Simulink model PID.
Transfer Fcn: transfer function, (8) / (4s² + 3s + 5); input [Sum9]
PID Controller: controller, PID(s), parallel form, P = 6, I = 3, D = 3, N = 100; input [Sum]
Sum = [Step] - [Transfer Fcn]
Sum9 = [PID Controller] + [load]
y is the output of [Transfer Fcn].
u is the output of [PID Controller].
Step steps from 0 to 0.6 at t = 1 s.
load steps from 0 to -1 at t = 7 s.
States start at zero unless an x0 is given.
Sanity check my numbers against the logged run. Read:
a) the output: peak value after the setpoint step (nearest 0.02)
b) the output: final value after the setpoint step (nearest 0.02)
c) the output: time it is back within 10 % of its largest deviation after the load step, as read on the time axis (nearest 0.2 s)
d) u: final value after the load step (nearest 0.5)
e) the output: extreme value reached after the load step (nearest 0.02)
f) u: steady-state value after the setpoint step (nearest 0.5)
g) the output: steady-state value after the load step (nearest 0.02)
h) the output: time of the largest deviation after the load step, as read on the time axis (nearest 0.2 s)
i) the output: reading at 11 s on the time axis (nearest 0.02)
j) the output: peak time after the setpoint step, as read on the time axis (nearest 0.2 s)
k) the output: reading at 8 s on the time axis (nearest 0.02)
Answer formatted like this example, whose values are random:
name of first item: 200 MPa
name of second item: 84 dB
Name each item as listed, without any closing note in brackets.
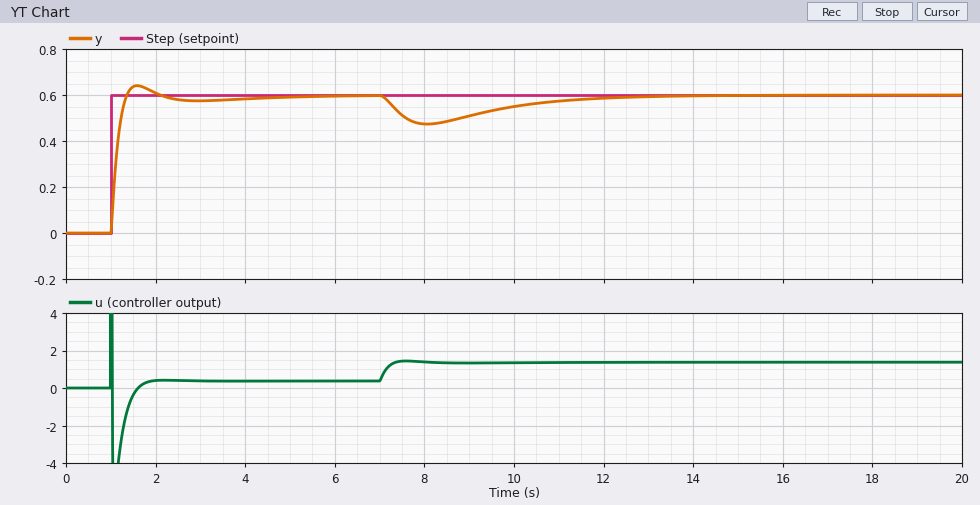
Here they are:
the output: peak value after the setpoint step: 0.64
the output: final value after the setpoint step: 0.60
the output: time it is back within 10 % of its largest deviation after the load step, as read on the time axis: 12.2 s
u: final value after the load step: 1.5
the output: extreme value reached after the load step: 0.48
u: steady-state value after the setpoint step: 0.5
the output: steady-state value after the load step: 0.60
the output: time of the largest deviation after the load step, as read on the time axis: 8.0 s
the output: reading at 11 s on the time axis: 0.58
the output: peak time after the setpoint step, as read on the time axis: 1.6 s
the output: reading at 8 s on the time axis: 0.48
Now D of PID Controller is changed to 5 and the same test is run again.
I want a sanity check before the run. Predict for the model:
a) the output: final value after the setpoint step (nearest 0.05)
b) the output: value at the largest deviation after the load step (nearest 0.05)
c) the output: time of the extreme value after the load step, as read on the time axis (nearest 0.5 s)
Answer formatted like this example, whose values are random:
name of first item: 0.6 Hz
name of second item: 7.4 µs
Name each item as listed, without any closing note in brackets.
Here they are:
the output: final value after the setpoint step: 0.60
the output: value at the largest deviation after the load step: 0.50
the output: time of the extreme value after the load step, as read on the time axis: 8.5 s
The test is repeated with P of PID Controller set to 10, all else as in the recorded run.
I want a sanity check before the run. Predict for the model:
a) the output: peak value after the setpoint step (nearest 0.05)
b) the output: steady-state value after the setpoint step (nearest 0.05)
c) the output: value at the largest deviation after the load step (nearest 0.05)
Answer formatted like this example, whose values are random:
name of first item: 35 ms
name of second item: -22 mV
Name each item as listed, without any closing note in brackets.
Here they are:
the output: peak value after the setpoint step: 0.70
the output: steady-state value after the setpoint step: 0.60
the output: value at the largest deviation after the load step: 0.50
